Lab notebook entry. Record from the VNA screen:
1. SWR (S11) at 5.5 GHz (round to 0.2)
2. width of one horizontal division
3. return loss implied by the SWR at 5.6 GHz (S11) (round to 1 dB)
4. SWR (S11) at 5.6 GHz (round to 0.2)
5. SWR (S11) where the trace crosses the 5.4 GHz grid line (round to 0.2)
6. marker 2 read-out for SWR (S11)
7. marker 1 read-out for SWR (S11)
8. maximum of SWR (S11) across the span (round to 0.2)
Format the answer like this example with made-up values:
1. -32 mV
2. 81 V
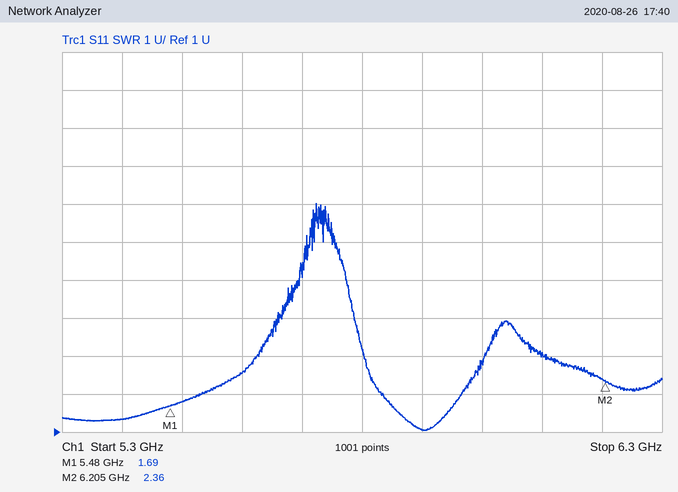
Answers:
1. 1.8
2. 100 MHz
3. 7 dB
4. 2.6
5. 1.4
6. 2.36
7. 1.69
8. 7.0
